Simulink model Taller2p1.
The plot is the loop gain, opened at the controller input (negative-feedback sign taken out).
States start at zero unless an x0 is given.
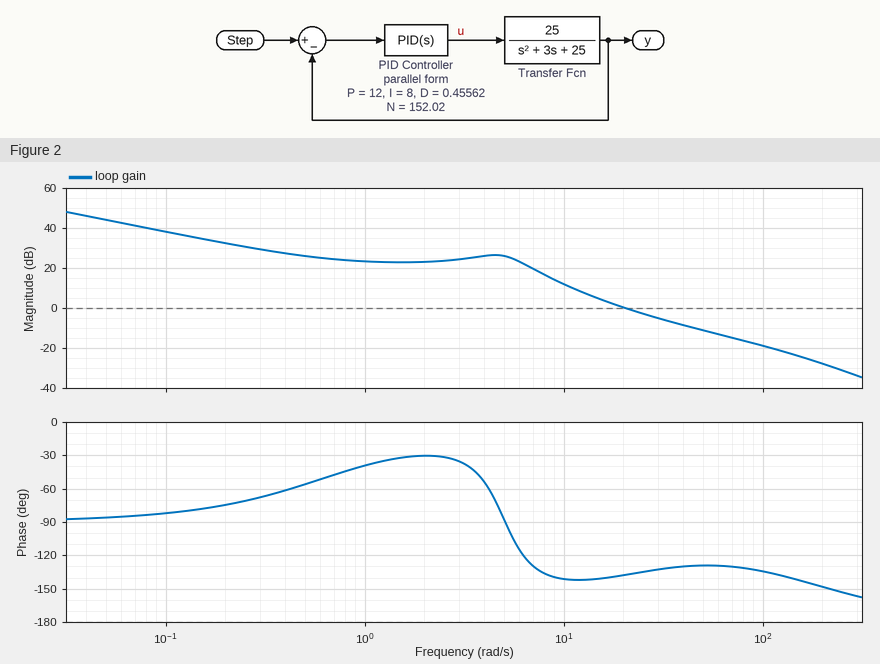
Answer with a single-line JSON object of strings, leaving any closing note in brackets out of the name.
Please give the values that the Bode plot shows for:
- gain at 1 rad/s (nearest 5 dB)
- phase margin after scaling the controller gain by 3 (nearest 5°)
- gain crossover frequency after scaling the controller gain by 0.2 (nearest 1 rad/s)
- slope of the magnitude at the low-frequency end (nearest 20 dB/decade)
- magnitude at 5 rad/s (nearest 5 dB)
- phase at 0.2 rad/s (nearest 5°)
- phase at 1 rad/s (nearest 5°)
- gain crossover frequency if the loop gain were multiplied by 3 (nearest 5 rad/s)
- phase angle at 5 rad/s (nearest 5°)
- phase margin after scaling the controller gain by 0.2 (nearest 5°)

{"gain at 1 rad/s": "25 dB", "phase margin after scaling the controller gain by 3": "50°", "gain crossover frequency after scaling the controller gain by 0.2": "9 rad/s", "slope of the magnitude at the low-frequency end": "-20 dB/decade", "magnitude at 5 rad/s": "25 dB", "phase at 0.2 rad/s": "-75°", "phase at 1 rad/s": "-40°", "gain crossover frequency if the loop gain were multiplied by 3": "45 rad/s", "phase angle at 5 rad/s": "-85°", "phase margin after scaling the controller gain by 0.2": "40°"}
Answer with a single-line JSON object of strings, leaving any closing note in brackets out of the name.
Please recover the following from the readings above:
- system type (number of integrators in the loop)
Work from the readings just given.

{"system type": "1"}
